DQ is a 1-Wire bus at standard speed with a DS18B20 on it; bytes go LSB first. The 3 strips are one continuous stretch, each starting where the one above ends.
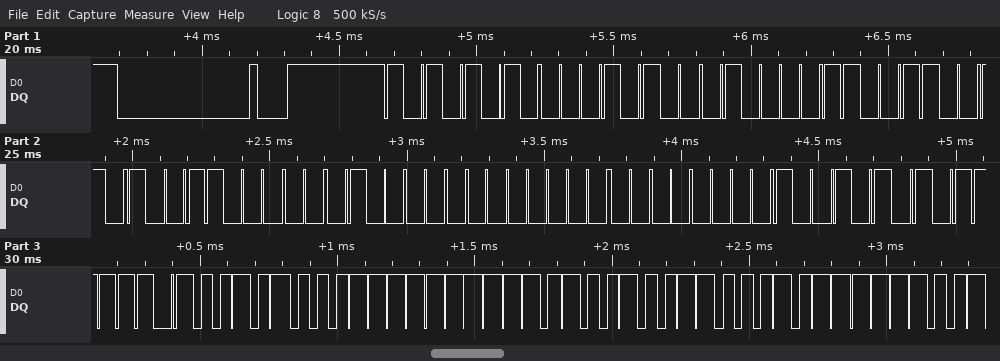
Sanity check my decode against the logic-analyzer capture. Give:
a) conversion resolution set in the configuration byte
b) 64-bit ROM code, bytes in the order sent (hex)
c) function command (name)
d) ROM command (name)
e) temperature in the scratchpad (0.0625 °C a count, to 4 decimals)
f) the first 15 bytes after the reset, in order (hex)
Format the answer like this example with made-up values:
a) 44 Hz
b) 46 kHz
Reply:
a) 10 bits
b) 28 C2 4C 19 08 00 00 A9
c) Read Scratchpad
d) Match ROM
e) -14.7500 °C
f) 55 28 C2 4C 19 08 00 00 A9 BE 14 FF 4B 46 3F
